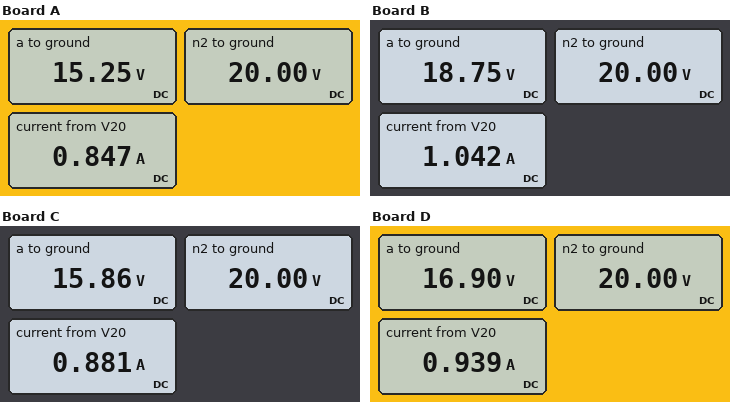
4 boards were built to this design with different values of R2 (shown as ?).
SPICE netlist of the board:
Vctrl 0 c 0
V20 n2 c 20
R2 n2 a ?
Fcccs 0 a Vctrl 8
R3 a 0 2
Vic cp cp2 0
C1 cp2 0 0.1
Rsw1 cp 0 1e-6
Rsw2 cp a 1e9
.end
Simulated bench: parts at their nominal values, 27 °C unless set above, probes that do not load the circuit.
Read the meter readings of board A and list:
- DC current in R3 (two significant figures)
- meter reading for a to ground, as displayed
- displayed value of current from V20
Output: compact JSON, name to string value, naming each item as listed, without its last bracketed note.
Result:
{"DC current in R3": "7.6 A", "meter reading for a to ground, as displayed": "15.25 V", "displayed value of current from V20": "0.847 A"}
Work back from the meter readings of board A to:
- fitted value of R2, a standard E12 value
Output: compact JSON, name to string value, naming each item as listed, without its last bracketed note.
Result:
{"fitted value of R2, a standard E12 value": "5.6 Ω"}
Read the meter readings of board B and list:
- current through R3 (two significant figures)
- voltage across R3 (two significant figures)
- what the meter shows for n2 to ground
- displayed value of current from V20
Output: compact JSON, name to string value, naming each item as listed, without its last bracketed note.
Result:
{"current through R3": "9.4 A", "voltage across R3": "19 V", "what the meter shows for n2 to ground": "20.00 V", "displayed value of current from V20": "1.042 A"}
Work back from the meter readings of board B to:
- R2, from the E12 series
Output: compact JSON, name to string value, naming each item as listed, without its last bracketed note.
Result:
{"R2, from the E12 series": "1.2 Ω"}
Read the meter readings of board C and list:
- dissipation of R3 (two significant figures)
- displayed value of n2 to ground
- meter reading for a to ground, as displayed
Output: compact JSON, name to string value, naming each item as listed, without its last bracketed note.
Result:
{"dissipation of R3": "130 W", "displayed value of n2 to ground": "20.00 V", "meter reading for a to ground, as displayed": "15.86 V"}
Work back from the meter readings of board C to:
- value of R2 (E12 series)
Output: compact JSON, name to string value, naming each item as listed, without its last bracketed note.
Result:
{"value of R2": "4.7 Ω"}
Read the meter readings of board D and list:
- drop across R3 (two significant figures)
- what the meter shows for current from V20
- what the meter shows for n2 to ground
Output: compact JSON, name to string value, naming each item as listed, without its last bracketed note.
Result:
{"drop across R3": "17 V", "what the meter shows for current from V20": "0.939 A", "what the meter shows for n2 to ground": "20.00 V"}
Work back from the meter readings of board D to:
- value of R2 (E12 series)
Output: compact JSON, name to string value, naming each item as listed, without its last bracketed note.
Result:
{"value of R2": "3.3 Ω"}
